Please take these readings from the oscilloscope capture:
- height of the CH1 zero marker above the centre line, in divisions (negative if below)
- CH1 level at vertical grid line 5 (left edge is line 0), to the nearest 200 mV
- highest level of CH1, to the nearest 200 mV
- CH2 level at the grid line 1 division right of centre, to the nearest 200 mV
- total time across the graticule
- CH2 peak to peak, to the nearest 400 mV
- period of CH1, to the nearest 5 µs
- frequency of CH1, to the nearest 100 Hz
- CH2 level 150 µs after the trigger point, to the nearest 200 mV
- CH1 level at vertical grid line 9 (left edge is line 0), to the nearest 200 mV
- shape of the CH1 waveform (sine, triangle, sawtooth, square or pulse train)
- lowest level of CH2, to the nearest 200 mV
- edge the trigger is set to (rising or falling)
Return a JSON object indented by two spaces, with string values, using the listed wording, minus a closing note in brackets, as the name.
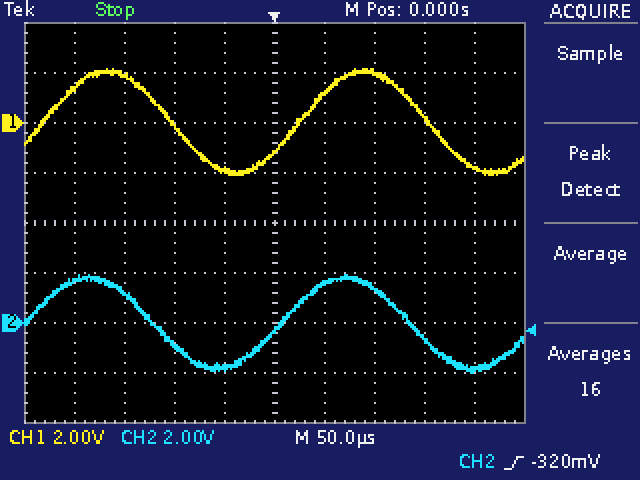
{
  "height of the CH1 zero marker above the centre line, in divisions": "+2.0 div",
  "CH1 level at vertical grid line 5 (left edge is line 0), to the nearest 200 mV": "-1.2 V",
  "highest level of CH1, to the nearest 200 mV": "2.2 V",
  "CH2 level at the grid line 1 division right of centre, to the nearest 200 mV": "1.6 V",
  "total time across the graticule": "500 µs",
  "CH2 peak to peak, to the nearest 400 mV": "4.0 V",
  "period of CH1, to the nearest 5 µs": "255 µs",
  "frequency of CH1, to the nearest 100 Hz": "3.9 kHz",
  "CH2 level 150 µs after the trigger point, to the nearest 200 mV": "-600 mV",
  "CH1 level at vertical grid line 9 (left edge is line 0), to the nearest 200 mV": "-1.8 V",
  "shape of the CH1 waveform": "sine",
  "lowest level of CH2, to the nearest 200 mV": "-2.0 V",
  "edge the trigger is set to": "rising"
}
